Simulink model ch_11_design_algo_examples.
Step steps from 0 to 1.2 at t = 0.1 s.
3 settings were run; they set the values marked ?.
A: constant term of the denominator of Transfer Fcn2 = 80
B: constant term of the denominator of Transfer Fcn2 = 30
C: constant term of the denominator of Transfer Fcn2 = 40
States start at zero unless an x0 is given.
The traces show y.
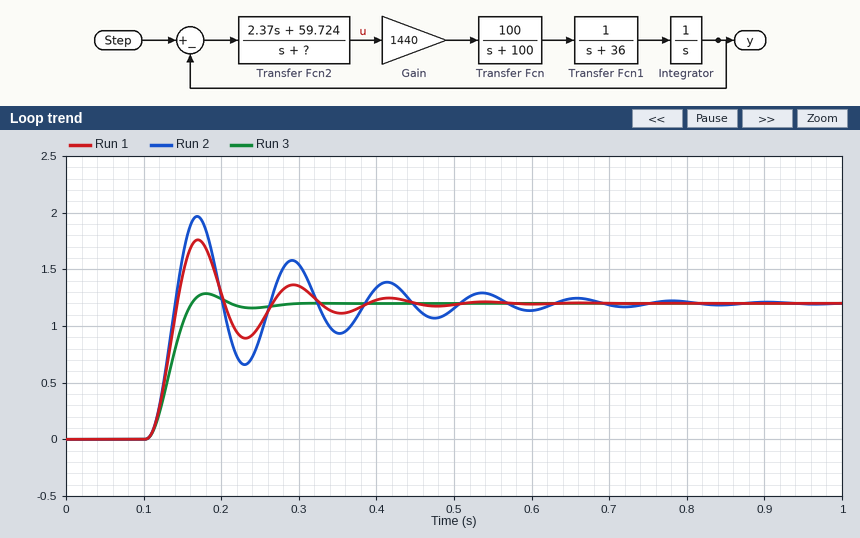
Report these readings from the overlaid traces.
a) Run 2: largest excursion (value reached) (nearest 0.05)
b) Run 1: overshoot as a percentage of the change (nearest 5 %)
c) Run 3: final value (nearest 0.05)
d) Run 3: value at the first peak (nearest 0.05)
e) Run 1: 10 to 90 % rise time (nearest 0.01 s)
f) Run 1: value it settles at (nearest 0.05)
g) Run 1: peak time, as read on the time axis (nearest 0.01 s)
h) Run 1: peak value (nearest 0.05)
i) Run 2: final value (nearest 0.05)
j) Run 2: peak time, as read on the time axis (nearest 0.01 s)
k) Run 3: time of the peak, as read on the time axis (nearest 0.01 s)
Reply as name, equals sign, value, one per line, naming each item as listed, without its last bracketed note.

Run 2: largest excursion (value reached) = 1.95
Run 1: overshoot as a percentage of the change = 45 %
Run 3: final value = 1.20
Run 3: value at the first peak = 1.30
Run 1: 10 to 90 % rise time = 0.03 s
Run 1: value it settles at = 1.20
Run 1: peak time, as read on the time axis = 0.17 s
Run 1: peak value = 1.75
Run 2: final value = 1.20
Run 2: peak time, as read on the time axis = 0.17 s
Run 3: time of the peak, as read on the time axis = 0.18 s
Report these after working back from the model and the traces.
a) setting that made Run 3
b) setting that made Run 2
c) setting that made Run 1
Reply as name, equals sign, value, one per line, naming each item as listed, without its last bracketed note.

setting that made Run 3 = A
setting that made Run 2 = B
setting that made Run 1 = C
